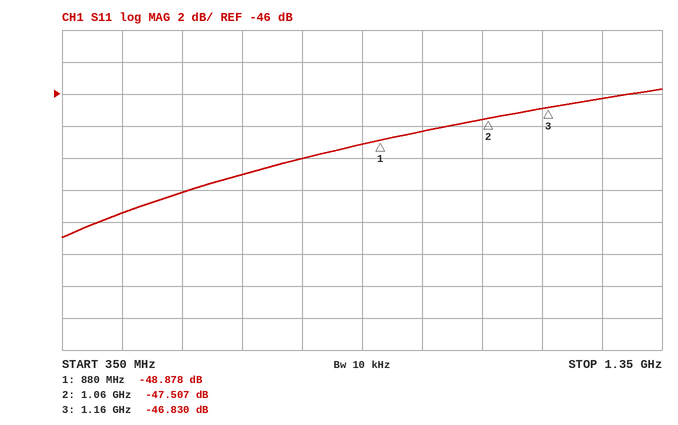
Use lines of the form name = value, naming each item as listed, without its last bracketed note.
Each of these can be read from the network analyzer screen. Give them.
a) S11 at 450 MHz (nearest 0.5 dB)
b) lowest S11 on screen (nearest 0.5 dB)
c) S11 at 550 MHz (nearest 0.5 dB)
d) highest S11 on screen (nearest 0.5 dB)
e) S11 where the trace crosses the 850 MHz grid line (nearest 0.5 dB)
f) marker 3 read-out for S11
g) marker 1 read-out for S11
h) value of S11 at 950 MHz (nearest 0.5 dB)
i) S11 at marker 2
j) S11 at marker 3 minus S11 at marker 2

S11 at 450 MHz = -53.5 dB
lowest S11 on screen = -55.0 dB
S11 at 550 MHz = -52.0 dB
highest S11 on screen = -45.5 dB
S11 where the trace crosses the 850 MHz grid line = -49.0 dB
marker 3 read-out for S11 = -46.830 dB
marker 1 read-out for S11 = -48.878 dB
value of S11 at 950 MHz = -48.5 dB
S11 at marker 2 = -47.507 dB
S11 at marker 3 minus S11 at marker 2 = 0.677 dB
